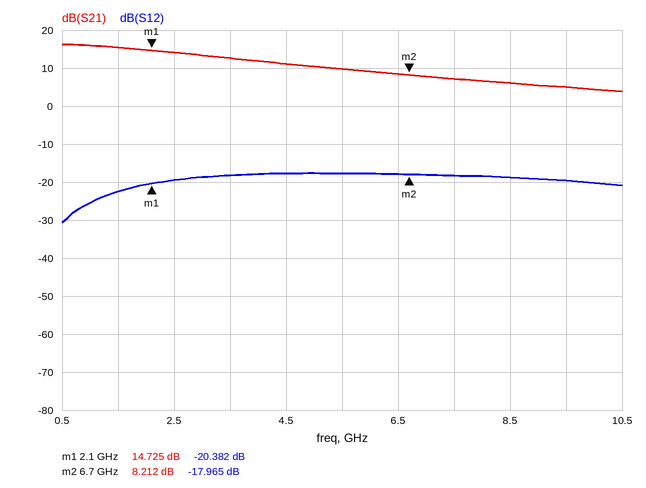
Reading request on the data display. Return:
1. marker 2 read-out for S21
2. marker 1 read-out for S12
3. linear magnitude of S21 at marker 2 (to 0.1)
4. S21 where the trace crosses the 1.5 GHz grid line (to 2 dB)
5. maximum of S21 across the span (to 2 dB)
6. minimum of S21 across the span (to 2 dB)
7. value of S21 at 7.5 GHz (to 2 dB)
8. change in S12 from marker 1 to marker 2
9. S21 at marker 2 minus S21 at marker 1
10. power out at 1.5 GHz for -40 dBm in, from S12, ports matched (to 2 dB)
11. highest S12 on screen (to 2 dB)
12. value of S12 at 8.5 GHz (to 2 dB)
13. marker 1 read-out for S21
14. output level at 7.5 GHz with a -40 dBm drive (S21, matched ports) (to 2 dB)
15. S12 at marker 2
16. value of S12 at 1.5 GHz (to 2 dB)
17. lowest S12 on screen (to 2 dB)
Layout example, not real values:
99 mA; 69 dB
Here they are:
8.212 dB; -20.382 dB; 2.6; 16 dB; 16 dB; 4 dB; 8 dB; 2.417 dB; -6.513 dB; -62 dBm; -18 dB; -18 dB; 14.725 dB; -32 dBm; -17.965 dB; -22 dB; -30 dB
